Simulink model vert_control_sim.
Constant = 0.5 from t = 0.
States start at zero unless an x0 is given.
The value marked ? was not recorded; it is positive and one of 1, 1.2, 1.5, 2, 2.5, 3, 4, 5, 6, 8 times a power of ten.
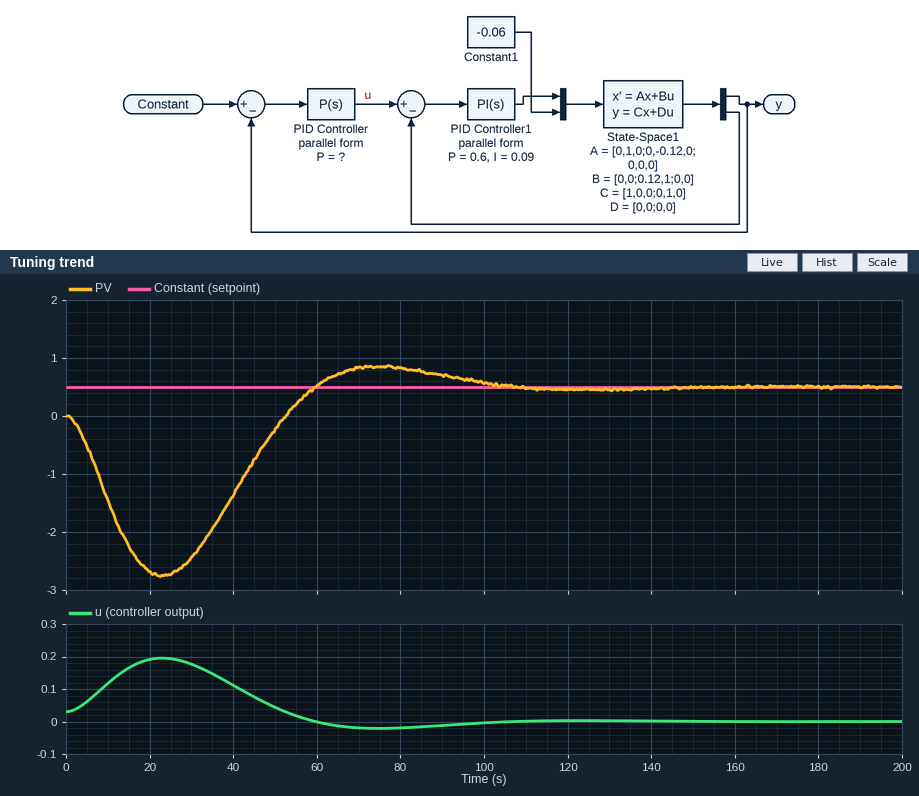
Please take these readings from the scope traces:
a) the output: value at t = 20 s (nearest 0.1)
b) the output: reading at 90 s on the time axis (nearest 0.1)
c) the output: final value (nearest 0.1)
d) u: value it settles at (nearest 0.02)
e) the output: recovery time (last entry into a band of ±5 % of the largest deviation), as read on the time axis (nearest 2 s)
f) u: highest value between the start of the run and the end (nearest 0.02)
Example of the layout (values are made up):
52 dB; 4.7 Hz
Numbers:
-2.7; 0.7; 0.5; 0.00; 94 s; 0.20
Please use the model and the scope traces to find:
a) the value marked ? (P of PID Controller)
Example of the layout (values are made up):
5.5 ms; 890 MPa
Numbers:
0.06
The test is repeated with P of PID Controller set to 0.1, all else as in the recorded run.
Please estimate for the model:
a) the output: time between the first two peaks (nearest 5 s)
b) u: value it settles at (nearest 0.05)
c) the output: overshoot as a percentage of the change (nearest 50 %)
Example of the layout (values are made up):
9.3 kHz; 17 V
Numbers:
70 s; 0.00; 100 %
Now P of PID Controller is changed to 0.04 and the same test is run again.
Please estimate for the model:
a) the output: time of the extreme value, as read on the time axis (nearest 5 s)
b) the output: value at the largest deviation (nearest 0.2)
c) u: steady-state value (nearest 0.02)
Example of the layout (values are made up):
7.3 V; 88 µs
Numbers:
25 s; -3.2; 0.00
